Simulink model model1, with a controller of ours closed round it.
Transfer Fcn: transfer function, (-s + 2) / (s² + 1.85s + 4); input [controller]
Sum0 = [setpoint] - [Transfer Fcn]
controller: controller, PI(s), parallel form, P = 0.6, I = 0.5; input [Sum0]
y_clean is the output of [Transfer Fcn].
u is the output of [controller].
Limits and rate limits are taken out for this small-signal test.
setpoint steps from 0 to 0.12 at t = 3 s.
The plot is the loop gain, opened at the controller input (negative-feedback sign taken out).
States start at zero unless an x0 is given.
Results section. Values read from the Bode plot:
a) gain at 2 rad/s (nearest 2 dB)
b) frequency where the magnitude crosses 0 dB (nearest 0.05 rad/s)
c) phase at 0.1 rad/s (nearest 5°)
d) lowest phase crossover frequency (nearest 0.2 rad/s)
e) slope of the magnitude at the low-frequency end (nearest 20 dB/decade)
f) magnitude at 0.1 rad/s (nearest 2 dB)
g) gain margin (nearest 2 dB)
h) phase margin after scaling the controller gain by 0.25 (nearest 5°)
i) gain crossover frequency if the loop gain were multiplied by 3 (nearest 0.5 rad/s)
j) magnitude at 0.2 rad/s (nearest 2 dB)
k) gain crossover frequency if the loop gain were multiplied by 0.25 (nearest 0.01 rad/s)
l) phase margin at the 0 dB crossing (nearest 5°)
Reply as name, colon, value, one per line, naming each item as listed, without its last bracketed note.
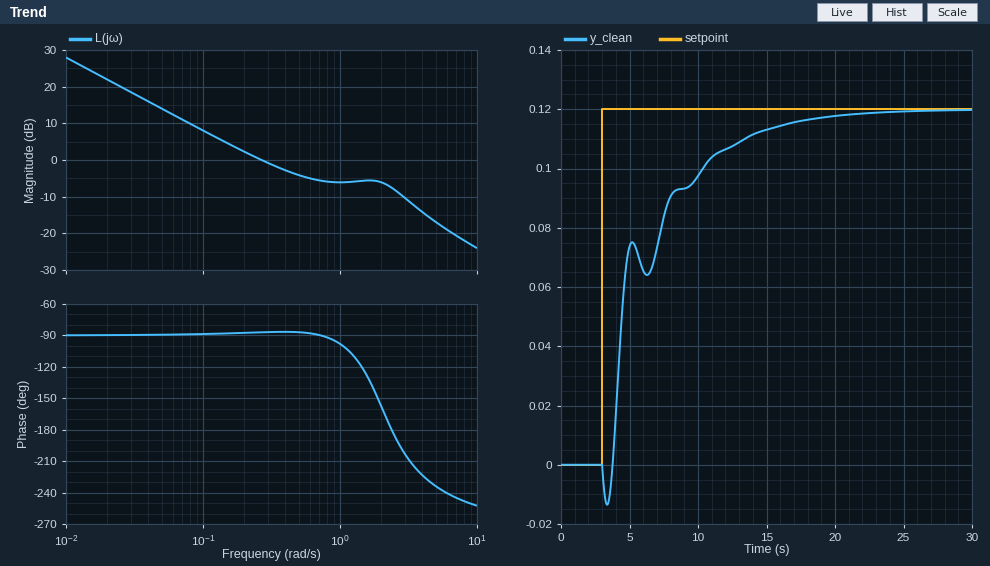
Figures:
gain at 2 rad/s: -6 dB
frequency where the magnitude crosses 0 dB: 0.25 rad/s
phase at 0.1 rad/s: -90°
lowest phase crossover frequency: 2.4 rad/s
slope of the magnitude at the low-frequency end: -20 dB/decade
magnitude at 0.1 rad/s: 8 dB
gain margin: 8 dB
phase margin after scaling the controller gain by 0.25: 90°
gain crossover frequency if the loop gain were multiplied by 3: 3.0 rad/s
magnitude at 0.2 rad/s: 2 dB
gain crossover frequency if the loop gain were multiplied by 0.25: 0.06 rad/s
phase margin at the 0 dB crossing: 95°
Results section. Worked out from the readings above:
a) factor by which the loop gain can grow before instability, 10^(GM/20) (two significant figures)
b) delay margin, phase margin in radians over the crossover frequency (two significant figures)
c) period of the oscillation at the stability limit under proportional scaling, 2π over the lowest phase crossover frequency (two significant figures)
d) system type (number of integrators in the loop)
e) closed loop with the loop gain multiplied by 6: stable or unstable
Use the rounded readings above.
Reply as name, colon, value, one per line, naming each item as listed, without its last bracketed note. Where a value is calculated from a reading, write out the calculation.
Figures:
factor by which the loop gain can grow before instability, 10^(GM/20): 10^(8 / 20) = 2.5
delay margin, phase margin in radians over the crossover frequency: 95 × π / 180 / 0.25 = 6.6 s
period of the oscillation at the stability limit under proportional scaling, 2π over the lowest phase crossover frequency: 2π / 2.4 = 2.6 s
system type: 1
closed loop with the loop gain multiplied by 6: stable or unstable: unstable
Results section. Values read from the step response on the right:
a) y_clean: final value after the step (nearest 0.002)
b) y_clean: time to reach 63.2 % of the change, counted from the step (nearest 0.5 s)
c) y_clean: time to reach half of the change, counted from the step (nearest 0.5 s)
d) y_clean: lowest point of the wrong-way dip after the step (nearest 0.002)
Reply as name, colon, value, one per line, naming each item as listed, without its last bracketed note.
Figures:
y_clean: final value after the step: 0.120
y_clean: time to reach 63.2 % of the change, counted from the step: 4.0 s
y_clean: time to reach half of the change, counted from the step: 1.5 s
y_clean: lowest point of the wrong-way dip after the step: -0.014
